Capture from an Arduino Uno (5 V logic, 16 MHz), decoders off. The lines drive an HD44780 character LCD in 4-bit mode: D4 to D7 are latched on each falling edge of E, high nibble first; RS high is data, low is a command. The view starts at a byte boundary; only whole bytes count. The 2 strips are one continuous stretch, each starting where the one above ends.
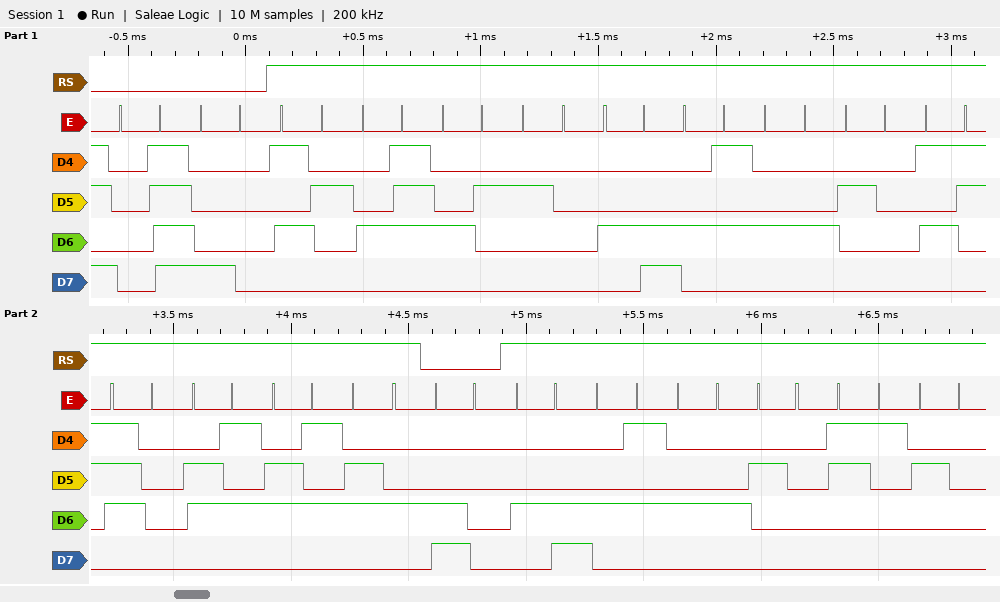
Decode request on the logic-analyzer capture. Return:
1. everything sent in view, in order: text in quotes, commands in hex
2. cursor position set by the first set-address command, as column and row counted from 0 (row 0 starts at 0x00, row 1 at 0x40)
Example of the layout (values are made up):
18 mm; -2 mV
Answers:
0x0F 0x80 "RGB LED Speed" 0xC0 "LED 1 "; column 0, row 0
